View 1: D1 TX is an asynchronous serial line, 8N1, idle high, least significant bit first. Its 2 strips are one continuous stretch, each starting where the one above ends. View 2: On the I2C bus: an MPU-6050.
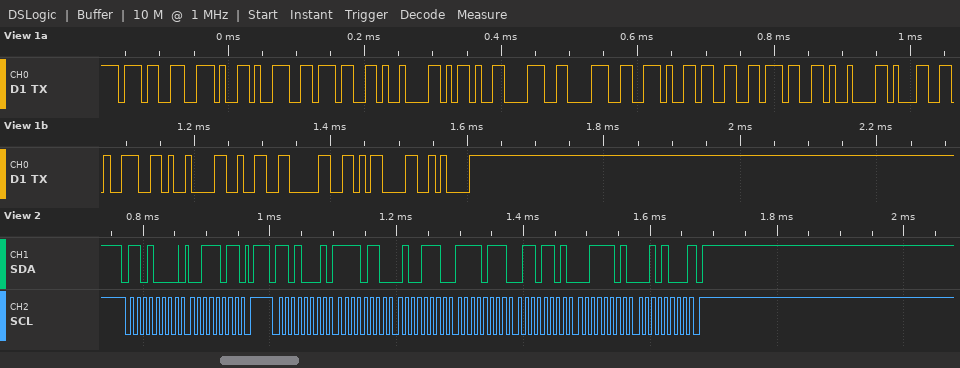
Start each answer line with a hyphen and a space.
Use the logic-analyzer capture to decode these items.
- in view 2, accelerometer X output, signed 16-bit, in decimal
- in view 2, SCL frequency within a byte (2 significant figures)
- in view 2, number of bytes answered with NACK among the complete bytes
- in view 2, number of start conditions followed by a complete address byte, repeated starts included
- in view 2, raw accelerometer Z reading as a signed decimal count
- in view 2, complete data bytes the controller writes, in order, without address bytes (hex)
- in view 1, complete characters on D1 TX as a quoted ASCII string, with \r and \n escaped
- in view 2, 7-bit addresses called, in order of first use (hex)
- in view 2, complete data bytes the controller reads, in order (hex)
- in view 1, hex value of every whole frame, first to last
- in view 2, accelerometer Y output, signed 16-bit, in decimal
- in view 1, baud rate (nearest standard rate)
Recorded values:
- -2482
- 100 kHz
- 1
- 2
- 15656
- 3B
- "7.97\t-88.37\t19\t20\r\n"
- 0x68
- F6 4E F7 6D 3D 28
- 0x37 0x2E 0x39 0x37 0x09 0x2D 0x38 0x38 0x2E 0x33 0x37 0x09 0x31 0x39 0x09 0x32 0x30 0x0D 0x0A
- -2195
- 115200 baud
